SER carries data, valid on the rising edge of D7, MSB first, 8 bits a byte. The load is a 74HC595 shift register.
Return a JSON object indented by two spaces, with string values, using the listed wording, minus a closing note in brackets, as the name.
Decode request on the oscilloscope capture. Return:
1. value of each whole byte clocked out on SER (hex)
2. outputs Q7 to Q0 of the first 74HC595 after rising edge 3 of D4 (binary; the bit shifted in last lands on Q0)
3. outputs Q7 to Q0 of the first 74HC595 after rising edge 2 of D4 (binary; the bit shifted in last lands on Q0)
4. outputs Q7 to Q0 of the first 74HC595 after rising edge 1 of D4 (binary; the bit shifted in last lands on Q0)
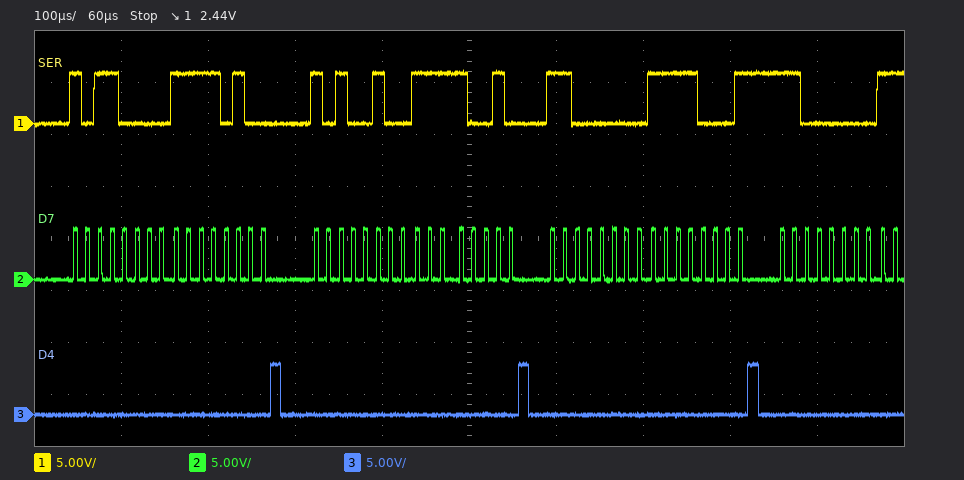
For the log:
{
  "value of each whole byte clocked out on SER": "B0 F4 A4 F2 C0 F1 C0",
  "outputs Q7 to Q0 of the first 74HC595 after rising edge 3 of D4": "11110001",
  "outputs Q7 to Q0 of the first 74HC595 after rising edge 2 of D4": "11110010",
  "outputs Q7 to Q0 of the first 74HC595 after rising edge 1 of D4": "11110100"
}
